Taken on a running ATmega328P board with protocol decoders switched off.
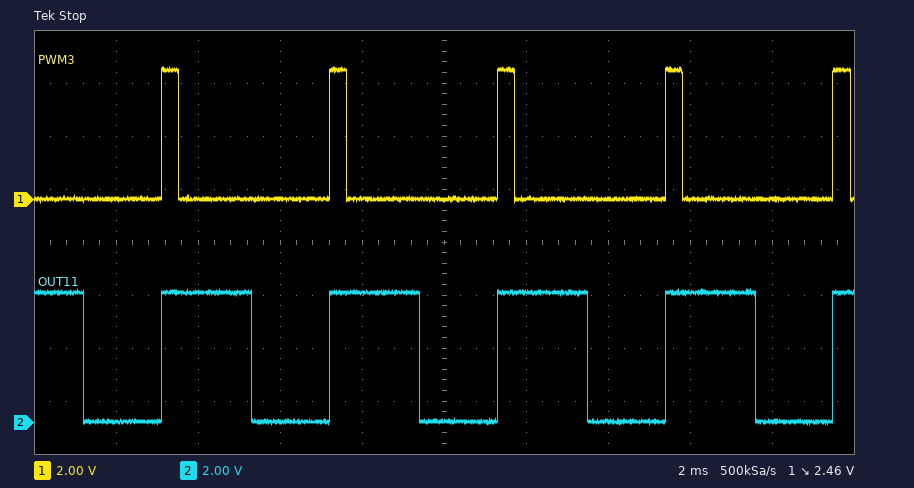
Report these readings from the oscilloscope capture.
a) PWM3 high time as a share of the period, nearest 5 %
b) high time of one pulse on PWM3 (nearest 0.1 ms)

10 %
0.4 ms
